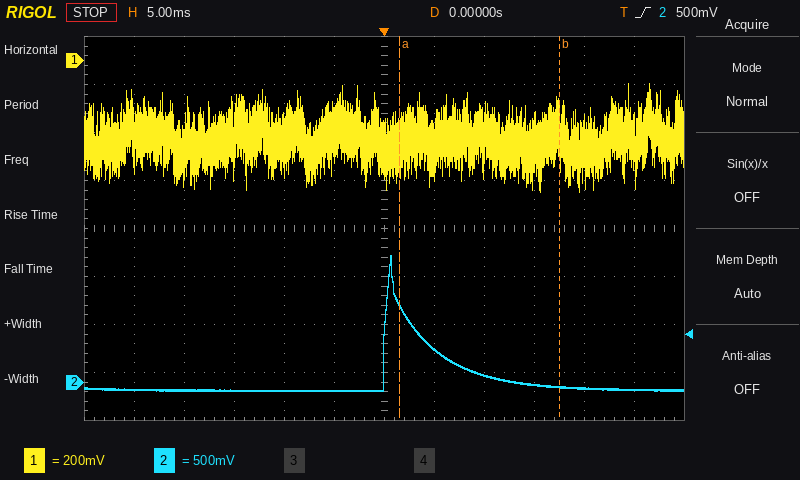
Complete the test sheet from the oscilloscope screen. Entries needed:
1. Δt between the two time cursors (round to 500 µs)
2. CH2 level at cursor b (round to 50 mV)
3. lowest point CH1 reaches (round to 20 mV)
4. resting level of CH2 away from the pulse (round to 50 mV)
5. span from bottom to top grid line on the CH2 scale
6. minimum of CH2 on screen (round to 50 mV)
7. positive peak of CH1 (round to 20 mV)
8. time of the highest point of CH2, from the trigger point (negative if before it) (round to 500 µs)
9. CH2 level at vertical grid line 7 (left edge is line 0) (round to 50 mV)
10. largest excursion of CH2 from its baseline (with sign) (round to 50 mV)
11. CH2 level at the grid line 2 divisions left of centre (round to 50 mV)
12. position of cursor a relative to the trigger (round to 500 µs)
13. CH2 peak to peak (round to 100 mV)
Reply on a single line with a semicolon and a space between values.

16.0 ms; -50 mV; -540 mV; -100 mV; 4 V; -100 mV; -100 mV; +500 µs; 350 mV; +1.40 V; -100 mV; +1.5 ms; 1.40 V
